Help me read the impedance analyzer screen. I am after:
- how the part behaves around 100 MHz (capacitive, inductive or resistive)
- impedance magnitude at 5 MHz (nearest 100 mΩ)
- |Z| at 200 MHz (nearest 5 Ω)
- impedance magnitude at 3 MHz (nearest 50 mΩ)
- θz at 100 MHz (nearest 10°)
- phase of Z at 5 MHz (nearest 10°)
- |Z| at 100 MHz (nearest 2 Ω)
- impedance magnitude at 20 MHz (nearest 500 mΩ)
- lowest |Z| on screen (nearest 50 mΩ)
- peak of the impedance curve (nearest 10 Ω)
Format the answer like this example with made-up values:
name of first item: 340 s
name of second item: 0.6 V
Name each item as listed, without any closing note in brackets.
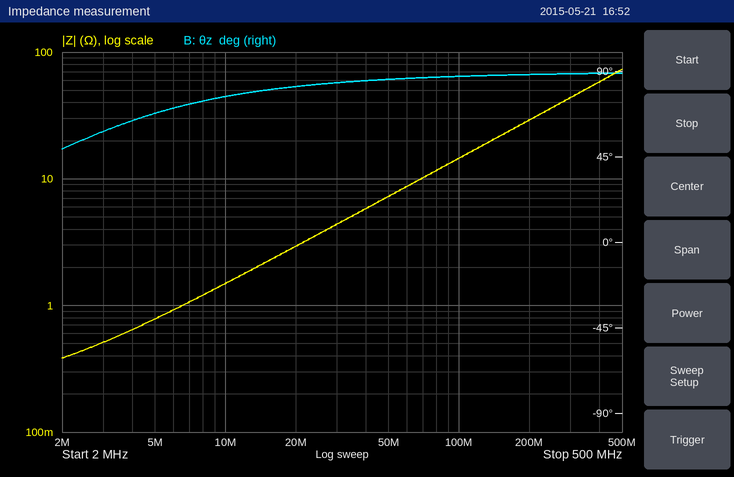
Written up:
how the part behaves around 100 MHz: inductive
impedance magnitude at 5 MHz: 800 mΩ
|Z| at 200 MHz: 30 Ω
impedance magnitude at 3 MHz: 500 mΩ
θz at 100 MHz: 90°
phase of Z at 5 MHz: 70°
|Z| at 100 MHz: 14 Ω
impedance magnitude at 20 MHz: 3.0 Ω
lowest |Z| on screen: 400 mΩ
peak of the impedance curve: 70 Ω
